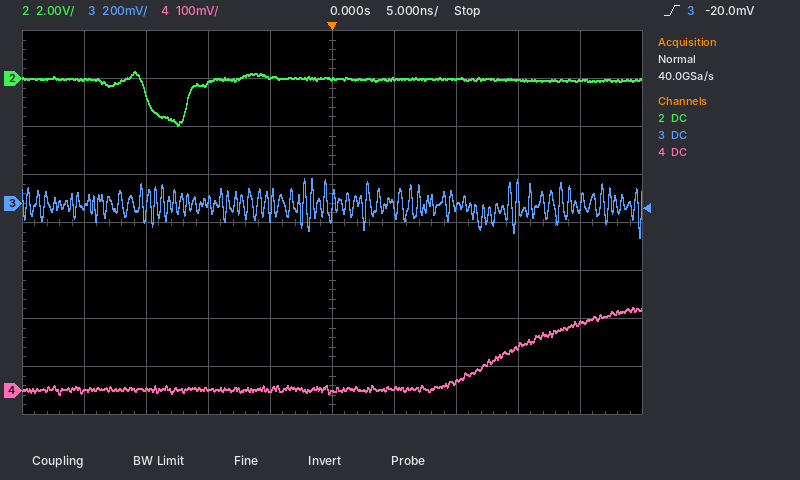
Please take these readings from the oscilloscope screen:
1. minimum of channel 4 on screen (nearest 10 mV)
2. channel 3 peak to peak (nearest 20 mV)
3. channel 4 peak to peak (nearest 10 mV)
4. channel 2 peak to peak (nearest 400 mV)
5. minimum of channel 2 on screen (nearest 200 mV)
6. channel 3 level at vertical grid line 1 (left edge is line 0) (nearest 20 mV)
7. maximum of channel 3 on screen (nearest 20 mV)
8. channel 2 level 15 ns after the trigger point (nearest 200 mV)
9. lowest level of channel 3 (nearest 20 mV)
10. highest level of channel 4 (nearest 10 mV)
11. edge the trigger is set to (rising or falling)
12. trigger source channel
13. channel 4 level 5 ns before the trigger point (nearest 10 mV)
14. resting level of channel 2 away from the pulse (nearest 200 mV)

-10 mV
240 mV
180 mV
2.4 V
-2.0 V
-20 mV
100 mV
0.0 V
-140 mV
170 mV
rising
channel 3
0 mV
0.0 V
